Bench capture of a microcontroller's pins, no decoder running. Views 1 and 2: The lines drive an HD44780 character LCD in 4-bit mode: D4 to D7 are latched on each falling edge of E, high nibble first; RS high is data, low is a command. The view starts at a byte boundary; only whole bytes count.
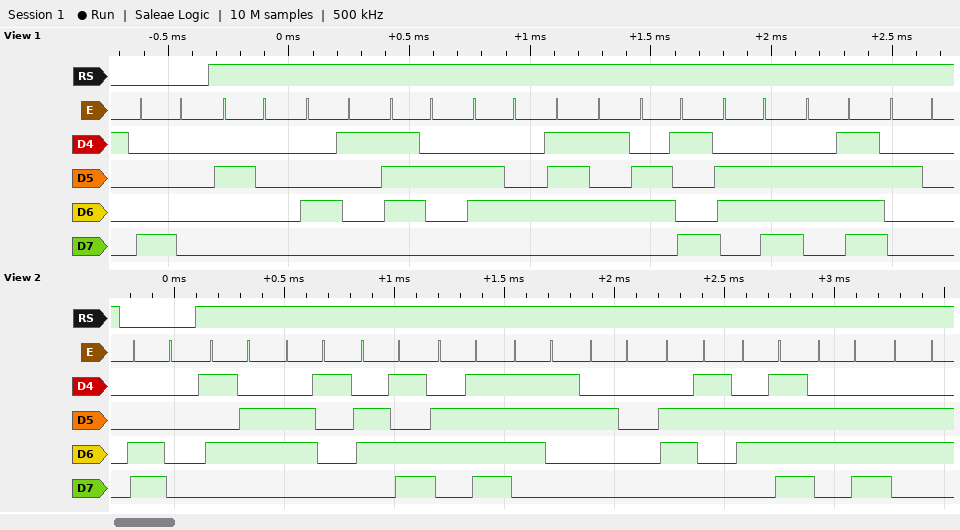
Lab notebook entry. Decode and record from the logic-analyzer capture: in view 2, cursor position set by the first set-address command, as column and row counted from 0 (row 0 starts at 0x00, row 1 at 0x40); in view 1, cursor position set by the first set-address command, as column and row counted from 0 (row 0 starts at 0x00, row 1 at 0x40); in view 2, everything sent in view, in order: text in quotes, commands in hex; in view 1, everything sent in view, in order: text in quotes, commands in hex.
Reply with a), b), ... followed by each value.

a) column 0, row 1
b) column 0, row 0
c) 0xC0 "Vamos conf"
d) 0x80 " Arduino "
